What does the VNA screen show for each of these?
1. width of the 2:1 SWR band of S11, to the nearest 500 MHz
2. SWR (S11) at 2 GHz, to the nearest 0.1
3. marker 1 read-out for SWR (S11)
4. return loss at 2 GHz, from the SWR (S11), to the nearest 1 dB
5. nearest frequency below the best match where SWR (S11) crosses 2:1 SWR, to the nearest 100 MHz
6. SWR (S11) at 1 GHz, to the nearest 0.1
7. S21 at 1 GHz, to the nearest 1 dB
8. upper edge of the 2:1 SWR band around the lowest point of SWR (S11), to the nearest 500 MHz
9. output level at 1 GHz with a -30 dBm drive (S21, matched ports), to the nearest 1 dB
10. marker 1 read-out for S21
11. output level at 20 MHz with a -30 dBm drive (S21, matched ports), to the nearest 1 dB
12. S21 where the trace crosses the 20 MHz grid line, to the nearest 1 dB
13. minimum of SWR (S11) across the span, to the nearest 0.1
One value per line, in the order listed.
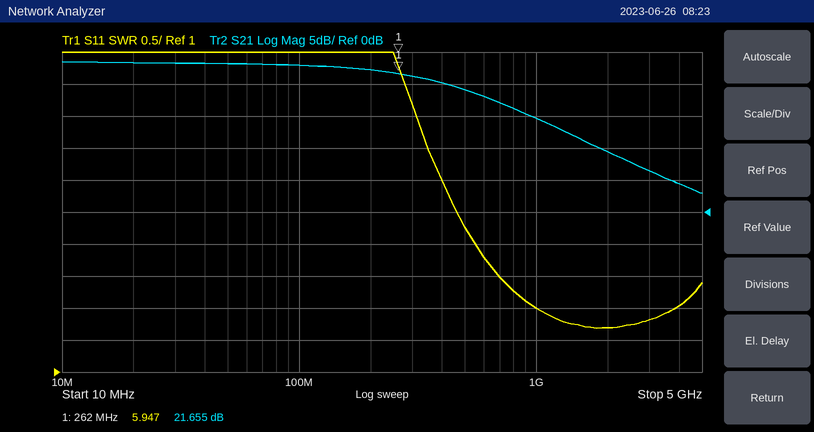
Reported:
3.0 GHz
1.7
5.947
12 dB
1.0 GHz
2.0
15 dB
4.0 GHz
-15 dBm
21.655 dB
-7 dBm
23 dB
1.7
